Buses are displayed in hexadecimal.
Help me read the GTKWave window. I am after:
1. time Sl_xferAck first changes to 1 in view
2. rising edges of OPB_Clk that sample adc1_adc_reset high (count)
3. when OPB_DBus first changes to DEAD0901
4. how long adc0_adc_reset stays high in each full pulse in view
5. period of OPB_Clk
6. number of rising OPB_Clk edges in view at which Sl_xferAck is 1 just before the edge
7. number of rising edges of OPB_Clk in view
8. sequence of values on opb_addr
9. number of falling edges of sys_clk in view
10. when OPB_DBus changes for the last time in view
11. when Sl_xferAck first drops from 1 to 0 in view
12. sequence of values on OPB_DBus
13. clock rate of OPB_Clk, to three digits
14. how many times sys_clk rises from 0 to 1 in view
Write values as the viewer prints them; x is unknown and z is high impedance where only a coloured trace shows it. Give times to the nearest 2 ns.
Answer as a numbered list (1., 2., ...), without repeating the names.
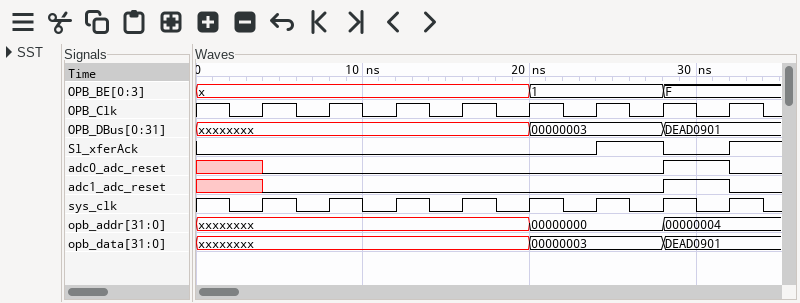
1. 24 ns
2. 1
3. 28 ns
4. 4 ns
5. 4 ns
6. 1
7. 8
8. xxxxxxxx, 00000000, 00000004
9. 9
10. 28 ns
11. 28 ns
12. xxxxxxxx, 00000003, DEAD0901
13. 250 MHz
14. 8
